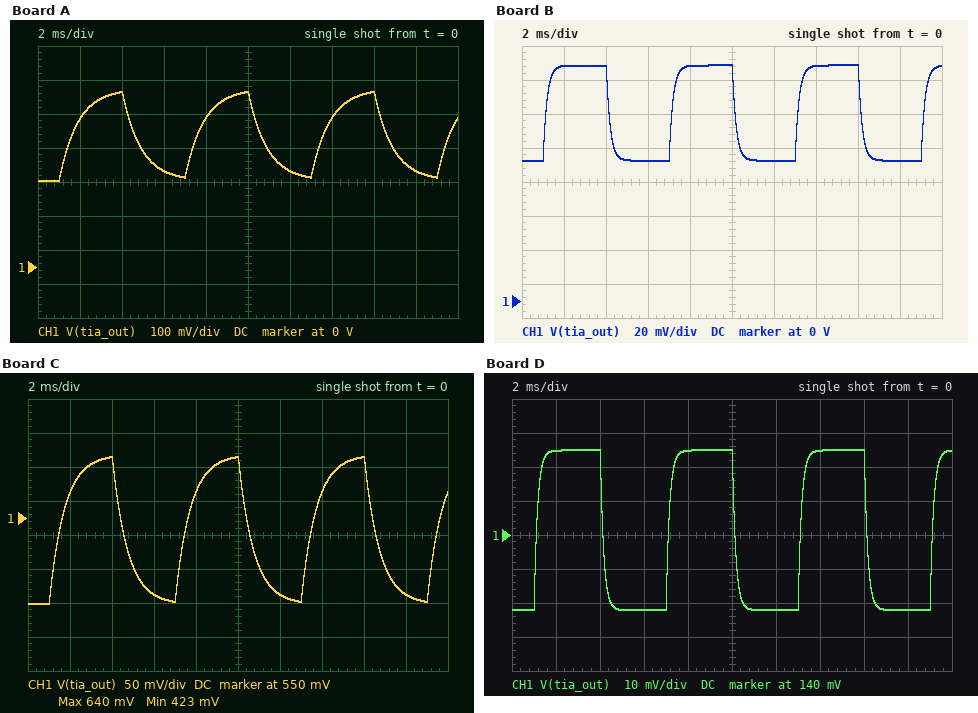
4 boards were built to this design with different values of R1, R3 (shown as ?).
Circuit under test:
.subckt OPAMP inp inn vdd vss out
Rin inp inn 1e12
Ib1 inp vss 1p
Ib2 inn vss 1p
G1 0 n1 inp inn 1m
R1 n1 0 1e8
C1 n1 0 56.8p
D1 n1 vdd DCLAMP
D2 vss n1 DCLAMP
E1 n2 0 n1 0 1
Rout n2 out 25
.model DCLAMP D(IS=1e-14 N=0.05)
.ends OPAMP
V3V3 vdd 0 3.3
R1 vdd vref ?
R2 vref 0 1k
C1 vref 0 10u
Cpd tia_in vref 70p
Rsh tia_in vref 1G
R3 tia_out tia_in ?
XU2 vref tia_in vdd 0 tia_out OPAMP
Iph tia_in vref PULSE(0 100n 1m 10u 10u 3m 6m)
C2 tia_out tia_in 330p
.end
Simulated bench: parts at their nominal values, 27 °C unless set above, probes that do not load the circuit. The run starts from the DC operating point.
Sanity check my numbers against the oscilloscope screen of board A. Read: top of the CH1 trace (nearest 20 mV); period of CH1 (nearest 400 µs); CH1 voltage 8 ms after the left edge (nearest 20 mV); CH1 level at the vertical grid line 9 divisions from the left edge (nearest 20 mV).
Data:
520 mV
6.0 ms
440 mV
280 mV
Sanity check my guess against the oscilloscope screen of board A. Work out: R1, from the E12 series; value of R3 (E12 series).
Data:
12 kΩ
2.7 MΩ
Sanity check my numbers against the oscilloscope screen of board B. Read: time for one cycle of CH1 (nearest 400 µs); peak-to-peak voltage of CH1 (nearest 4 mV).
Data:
6.0 ms
56 mV
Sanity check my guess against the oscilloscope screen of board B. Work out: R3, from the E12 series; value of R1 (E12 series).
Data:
560 kΩ
39 kΩ
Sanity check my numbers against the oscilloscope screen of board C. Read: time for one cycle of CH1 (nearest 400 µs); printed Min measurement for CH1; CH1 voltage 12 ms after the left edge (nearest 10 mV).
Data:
6.0 ms
423 mV
440 mV
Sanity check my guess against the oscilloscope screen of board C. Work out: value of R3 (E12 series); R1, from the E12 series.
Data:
2.2 MΩ
6.8 kΩ
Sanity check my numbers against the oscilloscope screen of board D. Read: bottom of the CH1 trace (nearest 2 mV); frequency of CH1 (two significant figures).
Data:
118 mV
170 Hz
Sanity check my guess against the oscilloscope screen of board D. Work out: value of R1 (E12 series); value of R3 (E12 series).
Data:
27 kΩ
470 kΩ
